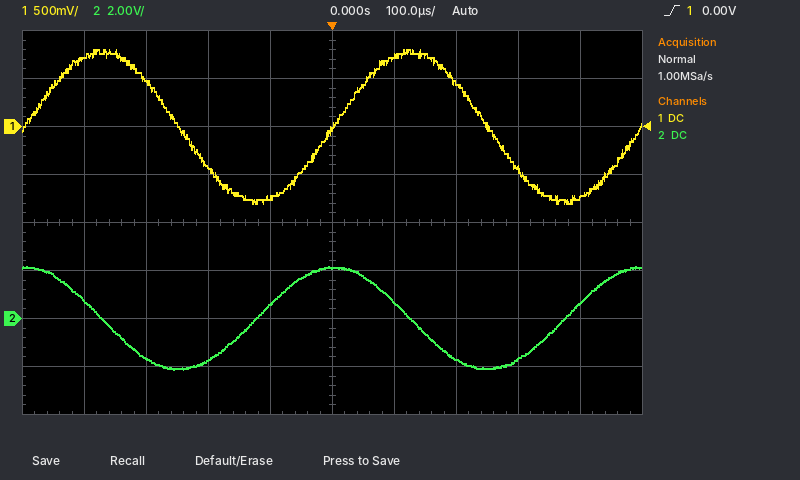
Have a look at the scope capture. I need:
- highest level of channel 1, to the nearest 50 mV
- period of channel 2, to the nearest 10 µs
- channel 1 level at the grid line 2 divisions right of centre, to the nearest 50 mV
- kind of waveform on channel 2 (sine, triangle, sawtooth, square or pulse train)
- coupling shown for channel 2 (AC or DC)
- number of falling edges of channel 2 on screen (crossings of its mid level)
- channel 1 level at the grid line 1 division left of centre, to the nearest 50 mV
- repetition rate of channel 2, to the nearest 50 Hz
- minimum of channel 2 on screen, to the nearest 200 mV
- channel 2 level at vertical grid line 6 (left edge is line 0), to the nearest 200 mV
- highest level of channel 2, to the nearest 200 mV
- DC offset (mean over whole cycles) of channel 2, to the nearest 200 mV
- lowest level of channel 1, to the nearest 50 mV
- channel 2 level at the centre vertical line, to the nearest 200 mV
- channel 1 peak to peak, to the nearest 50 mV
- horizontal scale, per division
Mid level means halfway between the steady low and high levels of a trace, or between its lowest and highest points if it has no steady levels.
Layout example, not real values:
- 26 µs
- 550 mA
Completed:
- 800 mV
- 500 µs
- 450 mV
- sine
- DC
- 2
- -750 mV
- 2.00 kHz
- -2.2 V
- 800 mV
- 2.2 V
- 0.0 V
- -800 mV
- 2.2 V
- 1.60 V
- 100 µs
